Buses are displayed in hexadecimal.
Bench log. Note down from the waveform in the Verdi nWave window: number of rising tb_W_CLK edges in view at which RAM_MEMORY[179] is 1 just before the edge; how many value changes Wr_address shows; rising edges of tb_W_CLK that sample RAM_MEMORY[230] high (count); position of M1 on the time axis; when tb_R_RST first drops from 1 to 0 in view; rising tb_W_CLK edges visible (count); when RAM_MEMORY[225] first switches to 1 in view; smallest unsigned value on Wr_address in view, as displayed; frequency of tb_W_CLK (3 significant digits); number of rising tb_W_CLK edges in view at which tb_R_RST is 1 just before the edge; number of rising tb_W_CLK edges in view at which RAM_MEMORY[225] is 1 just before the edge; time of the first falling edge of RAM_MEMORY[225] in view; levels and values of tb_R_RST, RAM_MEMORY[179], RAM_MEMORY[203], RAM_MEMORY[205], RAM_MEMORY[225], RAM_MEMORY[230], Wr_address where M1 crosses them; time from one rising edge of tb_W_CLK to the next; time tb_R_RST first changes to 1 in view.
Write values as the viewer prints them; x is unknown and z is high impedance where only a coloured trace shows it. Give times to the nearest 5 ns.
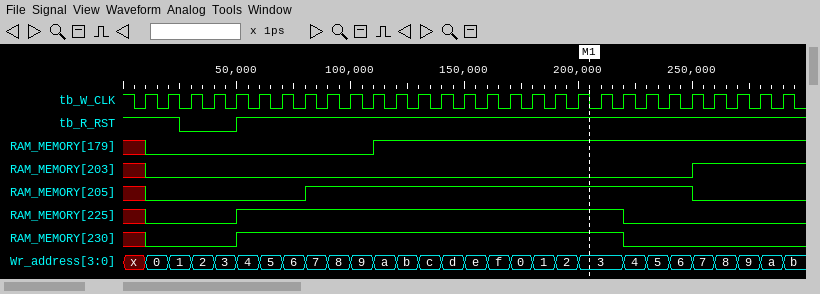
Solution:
18
28
17
205 ns
25 ns
29
50 ns
0
100 MHz
26
17
220 ns
tb_R_RST=1, RAM_MEMORY[179]=1, RAM_MEMORY[203]=0, RAM_MEMORY[205]=1, RAM_MEMORY[225]=1, RAM_MEMORY[230]=1, Wr_address=3
10 ns
50 ns
